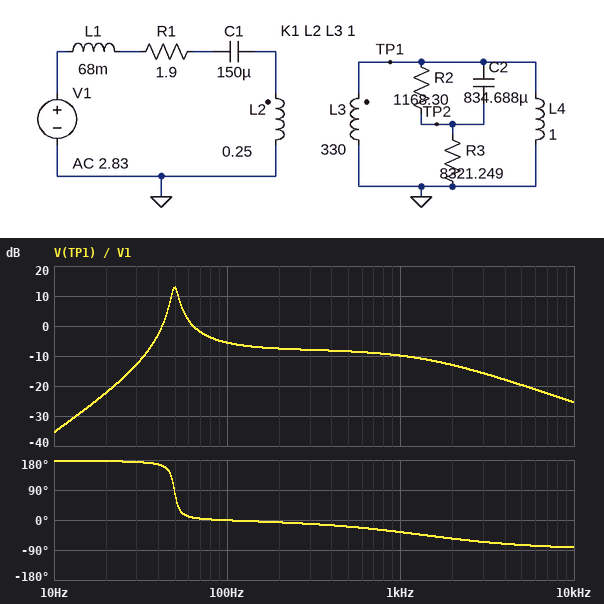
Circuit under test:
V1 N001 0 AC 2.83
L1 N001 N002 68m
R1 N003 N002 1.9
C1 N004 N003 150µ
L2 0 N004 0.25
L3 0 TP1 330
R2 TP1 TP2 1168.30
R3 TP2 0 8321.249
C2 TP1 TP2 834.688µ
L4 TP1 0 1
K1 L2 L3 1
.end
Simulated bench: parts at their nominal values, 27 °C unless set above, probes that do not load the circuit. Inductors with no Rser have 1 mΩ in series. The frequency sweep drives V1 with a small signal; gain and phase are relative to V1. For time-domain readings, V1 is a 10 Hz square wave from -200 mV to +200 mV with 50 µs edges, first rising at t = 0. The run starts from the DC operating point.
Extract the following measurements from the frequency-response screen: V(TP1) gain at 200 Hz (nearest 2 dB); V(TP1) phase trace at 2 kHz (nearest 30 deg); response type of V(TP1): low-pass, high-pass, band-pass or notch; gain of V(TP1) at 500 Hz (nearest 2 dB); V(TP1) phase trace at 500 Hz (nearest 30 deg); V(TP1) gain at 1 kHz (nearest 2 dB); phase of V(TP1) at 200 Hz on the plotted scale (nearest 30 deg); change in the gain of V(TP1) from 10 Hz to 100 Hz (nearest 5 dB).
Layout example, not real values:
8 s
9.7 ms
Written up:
-8 dB
-60 deg
band-pass
-8 dB
-30 deg
-10 dB
0 deg
30 dB
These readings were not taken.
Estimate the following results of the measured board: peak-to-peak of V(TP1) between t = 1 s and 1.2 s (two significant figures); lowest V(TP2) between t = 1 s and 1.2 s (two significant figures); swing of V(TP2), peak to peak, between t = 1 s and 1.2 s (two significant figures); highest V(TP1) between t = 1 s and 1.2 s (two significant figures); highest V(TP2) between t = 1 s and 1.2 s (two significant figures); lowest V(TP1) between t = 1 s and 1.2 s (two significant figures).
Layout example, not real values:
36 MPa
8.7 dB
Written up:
620 mV
-310 mV
620 mV
310 mV
310 mV
-310 mV
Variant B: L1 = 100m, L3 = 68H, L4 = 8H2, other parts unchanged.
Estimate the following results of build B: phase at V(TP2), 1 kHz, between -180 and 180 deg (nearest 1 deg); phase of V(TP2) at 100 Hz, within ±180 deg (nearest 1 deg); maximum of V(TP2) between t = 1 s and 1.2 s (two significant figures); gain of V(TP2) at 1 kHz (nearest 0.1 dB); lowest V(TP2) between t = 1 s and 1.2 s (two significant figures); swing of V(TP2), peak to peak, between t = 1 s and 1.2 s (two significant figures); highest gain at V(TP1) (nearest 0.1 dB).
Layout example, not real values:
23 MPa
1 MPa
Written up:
-77 deg
-21 deg
900 mV
-2.1 dB
-900 mV
1.8 V
30.2 dB
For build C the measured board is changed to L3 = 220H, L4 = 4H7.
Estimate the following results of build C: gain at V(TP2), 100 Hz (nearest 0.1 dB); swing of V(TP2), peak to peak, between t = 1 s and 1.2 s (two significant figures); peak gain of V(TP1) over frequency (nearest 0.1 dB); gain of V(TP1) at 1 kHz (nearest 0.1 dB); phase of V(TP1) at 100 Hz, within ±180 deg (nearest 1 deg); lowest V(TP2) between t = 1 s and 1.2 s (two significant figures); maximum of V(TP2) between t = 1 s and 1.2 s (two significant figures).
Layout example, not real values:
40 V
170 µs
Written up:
8.4 dB
2.4 V
26.6 dB
-4.0 dB
-14 deg
-1.2 V
1.2 V
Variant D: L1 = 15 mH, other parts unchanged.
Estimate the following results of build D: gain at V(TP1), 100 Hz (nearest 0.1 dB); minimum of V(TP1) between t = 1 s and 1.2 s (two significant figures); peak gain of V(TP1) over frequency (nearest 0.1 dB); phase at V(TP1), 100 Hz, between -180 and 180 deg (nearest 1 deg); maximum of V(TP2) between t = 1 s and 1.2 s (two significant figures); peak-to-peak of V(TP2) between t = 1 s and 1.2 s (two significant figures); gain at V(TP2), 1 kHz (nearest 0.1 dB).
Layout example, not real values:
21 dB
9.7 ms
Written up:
18.4 dB
-630 mV
19.3 dB
106 deg
630 mV
1.3 V
3.1 dB
